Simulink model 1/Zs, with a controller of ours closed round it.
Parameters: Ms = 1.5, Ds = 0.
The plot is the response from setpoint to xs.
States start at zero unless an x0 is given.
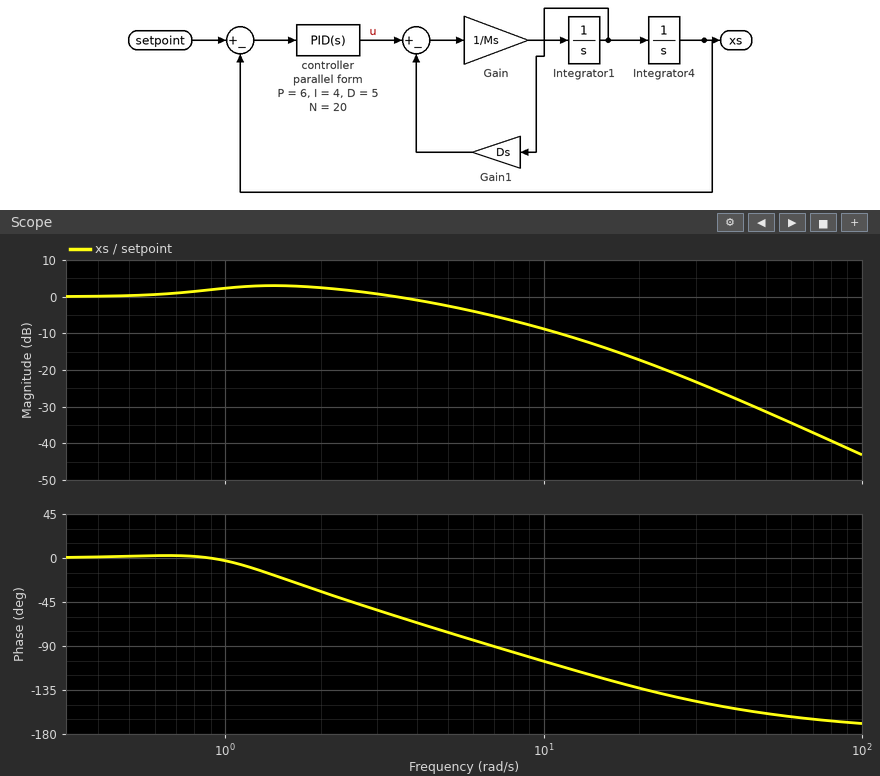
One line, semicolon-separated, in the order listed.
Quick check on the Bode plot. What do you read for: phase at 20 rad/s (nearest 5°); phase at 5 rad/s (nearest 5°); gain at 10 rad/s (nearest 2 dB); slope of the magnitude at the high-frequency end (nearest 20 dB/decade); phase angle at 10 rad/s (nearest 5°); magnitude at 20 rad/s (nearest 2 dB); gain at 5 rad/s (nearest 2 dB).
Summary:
-135°; -75°; -8 dB; -40 dB/decade; -105°; -18 dB; -2 dB
